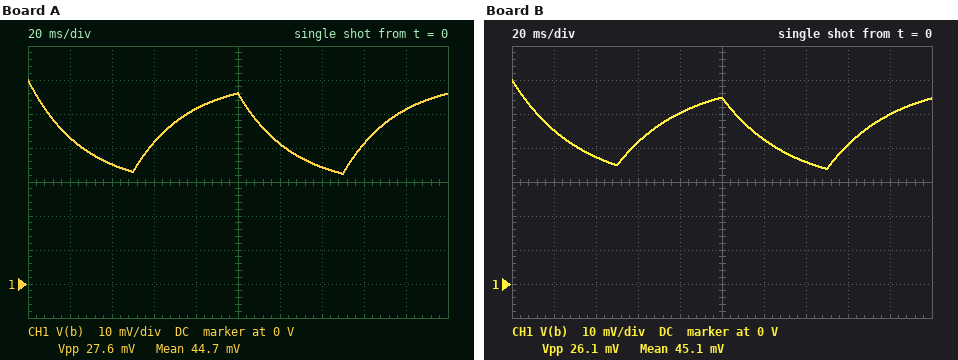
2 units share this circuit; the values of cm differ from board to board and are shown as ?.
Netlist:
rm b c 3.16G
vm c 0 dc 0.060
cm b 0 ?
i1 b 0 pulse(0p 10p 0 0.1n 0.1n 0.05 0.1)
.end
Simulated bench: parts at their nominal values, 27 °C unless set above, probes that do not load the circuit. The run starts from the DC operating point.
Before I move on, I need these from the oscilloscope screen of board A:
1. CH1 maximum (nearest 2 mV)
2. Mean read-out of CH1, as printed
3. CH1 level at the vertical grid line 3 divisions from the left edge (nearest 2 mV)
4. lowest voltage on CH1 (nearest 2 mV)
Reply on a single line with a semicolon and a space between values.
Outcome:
60 mV; 44.7 mV; 42 mV; 32 mV
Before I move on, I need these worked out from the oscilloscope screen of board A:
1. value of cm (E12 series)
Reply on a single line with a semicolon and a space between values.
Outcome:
8.2 pF
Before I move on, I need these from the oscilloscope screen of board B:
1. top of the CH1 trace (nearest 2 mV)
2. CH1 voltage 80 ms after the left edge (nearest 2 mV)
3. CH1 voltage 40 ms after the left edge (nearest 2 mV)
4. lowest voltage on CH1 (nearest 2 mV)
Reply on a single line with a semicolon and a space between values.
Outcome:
60 mV; 50 mV; 38 mV; 34 mV
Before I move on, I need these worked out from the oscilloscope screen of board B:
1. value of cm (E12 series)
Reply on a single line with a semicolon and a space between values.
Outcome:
10 pF
